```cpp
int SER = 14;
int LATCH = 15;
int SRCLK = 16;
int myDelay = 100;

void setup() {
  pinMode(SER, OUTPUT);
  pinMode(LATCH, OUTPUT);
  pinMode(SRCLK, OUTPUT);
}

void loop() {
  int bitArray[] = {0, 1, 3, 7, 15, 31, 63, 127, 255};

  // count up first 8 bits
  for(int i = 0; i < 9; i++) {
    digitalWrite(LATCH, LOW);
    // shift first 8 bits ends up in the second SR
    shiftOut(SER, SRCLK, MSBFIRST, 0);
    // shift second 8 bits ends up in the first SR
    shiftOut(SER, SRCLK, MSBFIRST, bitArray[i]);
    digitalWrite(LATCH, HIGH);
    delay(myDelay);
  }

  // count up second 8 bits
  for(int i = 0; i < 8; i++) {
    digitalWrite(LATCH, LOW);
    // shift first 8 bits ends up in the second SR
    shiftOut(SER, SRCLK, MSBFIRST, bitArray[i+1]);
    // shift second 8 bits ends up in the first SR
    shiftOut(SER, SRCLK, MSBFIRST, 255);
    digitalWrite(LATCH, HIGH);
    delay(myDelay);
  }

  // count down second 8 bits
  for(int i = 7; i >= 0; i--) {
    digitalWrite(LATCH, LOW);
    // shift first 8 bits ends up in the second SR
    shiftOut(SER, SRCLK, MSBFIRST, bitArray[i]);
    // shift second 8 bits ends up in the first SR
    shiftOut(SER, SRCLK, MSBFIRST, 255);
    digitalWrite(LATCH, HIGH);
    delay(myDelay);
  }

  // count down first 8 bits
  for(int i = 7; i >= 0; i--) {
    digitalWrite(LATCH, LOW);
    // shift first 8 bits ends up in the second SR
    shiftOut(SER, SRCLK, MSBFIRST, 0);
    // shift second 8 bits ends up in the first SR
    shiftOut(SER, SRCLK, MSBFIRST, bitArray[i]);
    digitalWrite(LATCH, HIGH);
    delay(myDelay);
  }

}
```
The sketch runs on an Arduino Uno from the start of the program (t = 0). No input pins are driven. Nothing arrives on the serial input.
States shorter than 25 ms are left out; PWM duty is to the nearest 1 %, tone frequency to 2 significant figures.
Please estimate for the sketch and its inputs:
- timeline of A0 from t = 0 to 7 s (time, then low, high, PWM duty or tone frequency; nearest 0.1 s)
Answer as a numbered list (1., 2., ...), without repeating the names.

1. 0 s low; 0.1 s high; 3.2 s low; 3.4 s high; 6.5 s low; 6.7 s high
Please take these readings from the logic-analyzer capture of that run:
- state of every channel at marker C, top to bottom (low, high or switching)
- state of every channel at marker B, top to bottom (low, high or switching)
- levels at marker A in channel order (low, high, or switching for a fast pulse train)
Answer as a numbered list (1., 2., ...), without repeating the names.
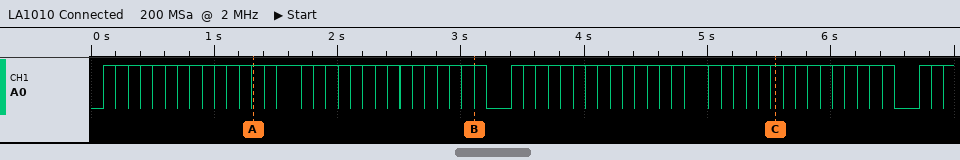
1. A0 high
2. A0 high
3. A0 high
